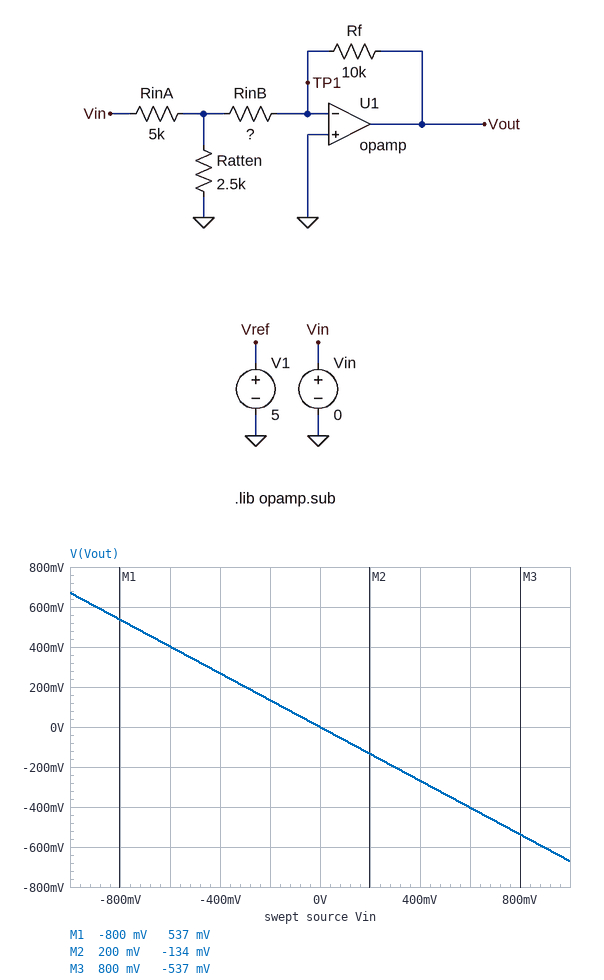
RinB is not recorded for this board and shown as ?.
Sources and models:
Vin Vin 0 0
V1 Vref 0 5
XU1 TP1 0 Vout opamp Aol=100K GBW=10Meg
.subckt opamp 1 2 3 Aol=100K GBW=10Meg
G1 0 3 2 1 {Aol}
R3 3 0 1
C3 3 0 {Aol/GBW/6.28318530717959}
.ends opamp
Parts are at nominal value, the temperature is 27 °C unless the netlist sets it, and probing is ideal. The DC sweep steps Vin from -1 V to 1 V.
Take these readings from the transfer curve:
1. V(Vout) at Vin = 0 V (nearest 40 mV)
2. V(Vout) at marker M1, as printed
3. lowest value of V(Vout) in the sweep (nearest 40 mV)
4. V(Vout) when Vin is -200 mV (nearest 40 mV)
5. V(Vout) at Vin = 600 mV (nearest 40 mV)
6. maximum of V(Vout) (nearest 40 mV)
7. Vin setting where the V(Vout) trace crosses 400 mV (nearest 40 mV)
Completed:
0 V
537 mV
-680 mV
120 mV
-400 mV
680 mV
-600 mV
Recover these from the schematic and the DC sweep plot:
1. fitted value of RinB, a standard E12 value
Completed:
3.3 kΩ
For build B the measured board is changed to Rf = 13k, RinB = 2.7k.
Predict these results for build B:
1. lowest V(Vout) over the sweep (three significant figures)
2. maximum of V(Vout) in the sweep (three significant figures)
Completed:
-992 mV
992 mV
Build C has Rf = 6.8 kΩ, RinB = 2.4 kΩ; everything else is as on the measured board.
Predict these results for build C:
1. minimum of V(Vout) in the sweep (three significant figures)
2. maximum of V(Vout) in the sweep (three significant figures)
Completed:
-557 mV
557 mV
